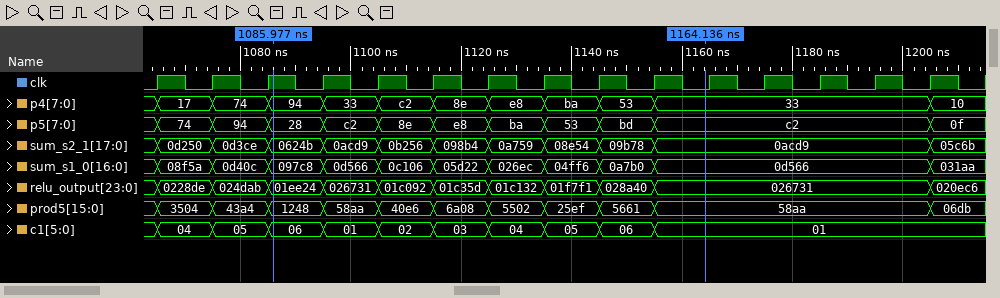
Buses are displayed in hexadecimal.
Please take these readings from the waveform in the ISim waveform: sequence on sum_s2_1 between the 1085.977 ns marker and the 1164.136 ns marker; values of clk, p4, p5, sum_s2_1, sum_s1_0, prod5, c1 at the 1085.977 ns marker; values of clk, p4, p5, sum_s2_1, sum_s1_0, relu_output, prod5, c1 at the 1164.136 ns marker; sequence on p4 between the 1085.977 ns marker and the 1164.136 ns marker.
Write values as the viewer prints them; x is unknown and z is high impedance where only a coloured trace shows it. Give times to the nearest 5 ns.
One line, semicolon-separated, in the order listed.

0624b, 0acd9, 0b256, 098b4, 0a759, 08e54, 09b78, 0acd9; clk=1, p4=94, p5=28, sum_s2_1=0624b, sum_s1_0=097c8, prod5=1248, c1=06; clk=0, p4=33, p5=c2, sum_s2_1=0acd9, sum_s1_0=0d566, relu_output=026731, prod5=58aa, c1=01; 94, 33, c2, 8e, e8, ba, 53, 33
